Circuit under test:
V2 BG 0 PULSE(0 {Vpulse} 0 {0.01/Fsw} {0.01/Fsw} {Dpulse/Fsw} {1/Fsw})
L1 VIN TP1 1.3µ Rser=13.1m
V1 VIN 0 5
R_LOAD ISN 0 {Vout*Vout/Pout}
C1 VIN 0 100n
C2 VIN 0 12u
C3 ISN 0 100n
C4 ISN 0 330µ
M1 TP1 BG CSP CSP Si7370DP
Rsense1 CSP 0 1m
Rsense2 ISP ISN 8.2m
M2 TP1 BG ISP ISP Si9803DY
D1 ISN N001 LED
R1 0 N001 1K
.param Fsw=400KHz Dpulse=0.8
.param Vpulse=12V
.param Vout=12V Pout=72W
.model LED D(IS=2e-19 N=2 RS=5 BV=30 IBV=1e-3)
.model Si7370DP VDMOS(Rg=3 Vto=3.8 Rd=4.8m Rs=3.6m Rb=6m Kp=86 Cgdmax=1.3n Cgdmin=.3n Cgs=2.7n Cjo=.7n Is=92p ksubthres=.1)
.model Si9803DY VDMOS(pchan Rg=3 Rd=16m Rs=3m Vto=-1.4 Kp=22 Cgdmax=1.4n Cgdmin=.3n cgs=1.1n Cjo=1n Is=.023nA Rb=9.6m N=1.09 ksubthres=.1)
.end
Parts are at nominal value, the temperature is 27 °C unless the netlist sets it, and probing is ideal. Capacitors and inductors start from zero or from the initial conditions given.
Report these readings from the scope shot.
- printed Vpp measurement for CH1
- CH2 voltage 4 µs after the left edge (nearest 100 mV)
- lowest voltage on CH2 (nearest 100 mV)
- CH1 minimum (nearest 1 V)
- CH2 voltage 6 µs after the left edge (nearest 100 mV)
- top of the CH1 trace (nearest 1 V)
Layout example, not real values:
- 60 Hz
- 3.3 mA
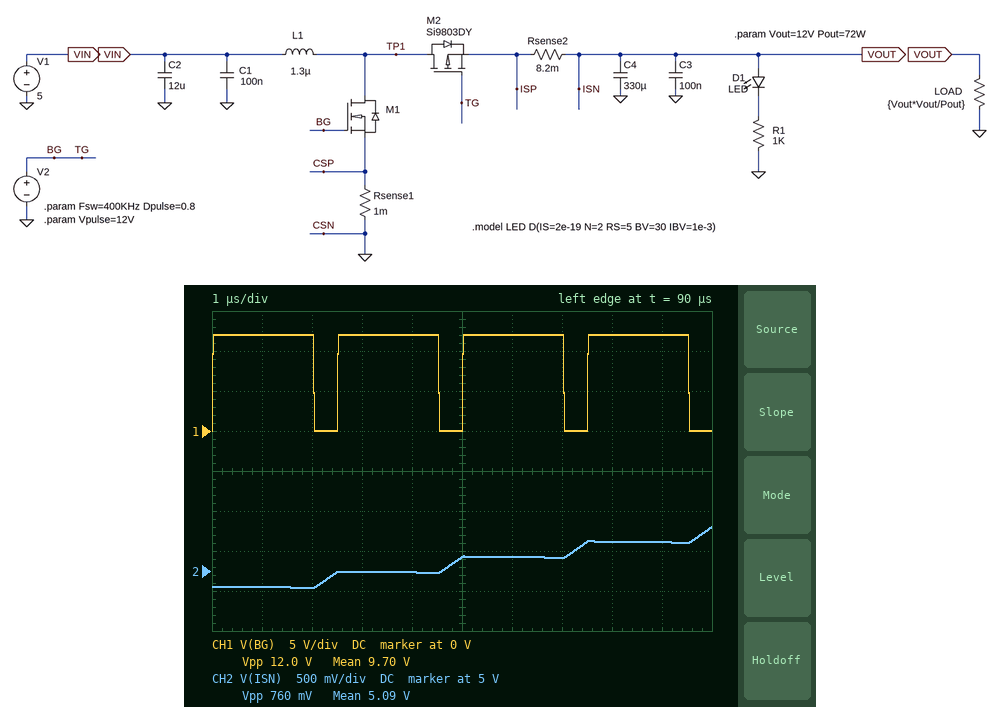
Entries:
- 12.0 V
- 5.0 V
- 4.8 V
- 0 V
- 5.2 V
- 12 V
